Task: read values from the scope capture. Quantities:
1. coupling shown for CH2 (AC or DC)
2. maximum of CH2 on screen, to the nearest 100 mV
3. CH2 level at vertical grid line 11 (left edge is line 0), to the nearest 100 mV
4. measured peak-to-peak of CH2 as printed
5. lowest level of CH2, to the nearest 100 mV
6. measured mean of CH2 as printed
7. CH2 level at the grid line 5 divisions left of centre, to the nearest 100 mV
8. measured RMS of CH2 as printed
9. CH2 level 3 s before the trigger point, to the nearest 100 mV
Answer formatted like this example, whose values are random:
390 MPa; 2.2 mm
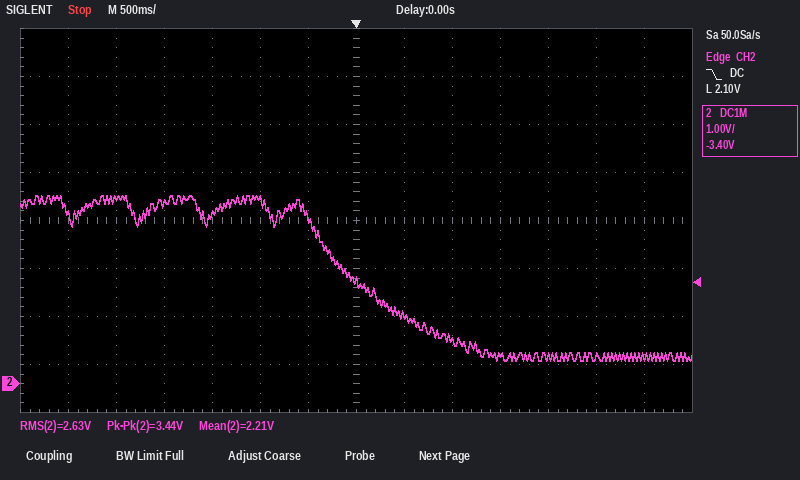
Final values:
DC; 3.9 V; 600 mV; 3.44 V; 500 mV; 2.21 V; 3.9 V; 2.63 V; 3.5 V
